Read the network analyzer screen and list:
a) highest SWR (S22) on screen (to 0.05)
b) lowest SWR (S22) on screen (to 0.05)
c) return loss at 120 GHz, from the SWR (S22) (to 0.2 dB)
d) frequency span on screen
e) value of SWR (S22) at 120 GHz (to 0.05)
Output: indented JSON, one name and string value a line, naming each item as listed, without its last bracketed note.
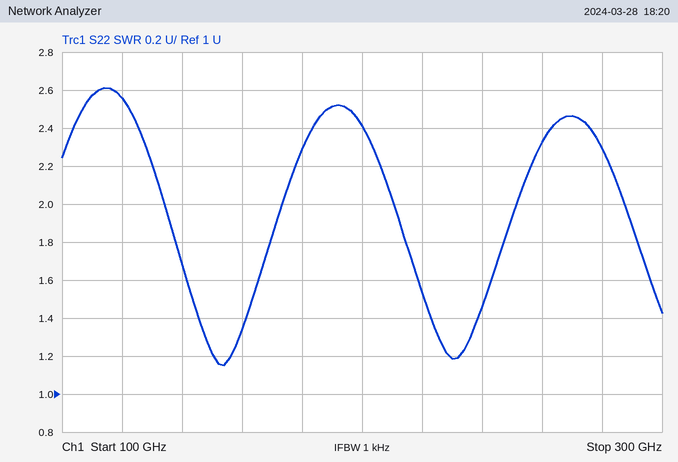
{
  "highest SWR (S22) on screen": "2.60",
  "lowest SWR (S22) on screen": "1.15",
  "return loss at 120 GHz, from the SWR (S22)": "7.2 dB",
  "frequency span on screen": "200 GHz",
  "value of SWR (S22) at 120 GHz": "2.55"
}
